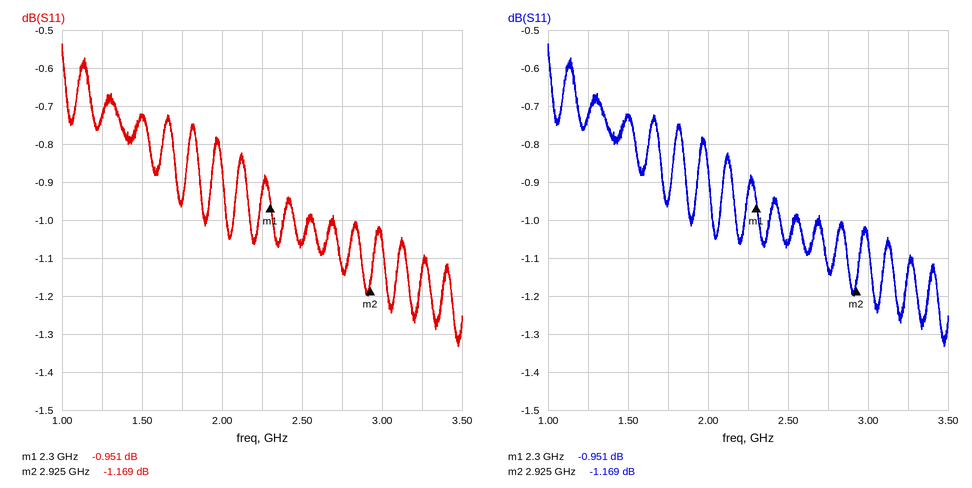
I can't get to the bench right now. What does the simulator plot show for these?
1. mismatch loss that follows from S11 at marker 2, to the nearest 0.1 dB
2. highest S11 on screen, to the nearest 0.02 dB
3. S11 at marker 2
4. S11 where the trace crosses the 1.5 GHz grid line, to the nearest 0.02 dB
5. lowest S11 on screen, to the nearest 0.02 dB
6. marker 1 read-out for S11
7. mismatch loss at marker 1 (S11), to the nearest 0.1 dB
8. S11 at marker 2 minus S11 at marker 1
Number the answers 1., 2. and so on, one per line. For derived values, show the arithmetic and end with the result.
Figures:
1. −10 log10(1 − 10^(-1.169/10)) ≈ 6.3 dB
2. -0.54 dB
3. -1.169 dB
4. -0.72 dB
5. -1.34 dB
6. -0.951 dB
7. −10 log10(1 − 10^(-0.951/10)) ≈ 7.1 dB
8. -1.169 − (-0.951) = -0.218 dB
